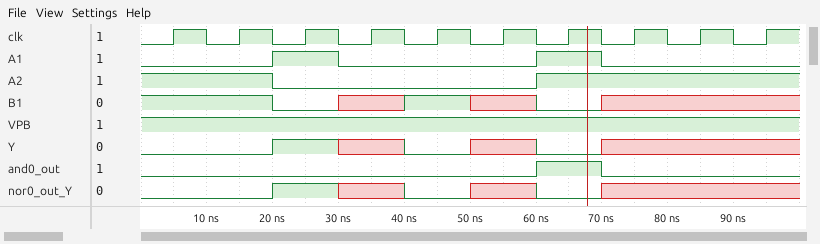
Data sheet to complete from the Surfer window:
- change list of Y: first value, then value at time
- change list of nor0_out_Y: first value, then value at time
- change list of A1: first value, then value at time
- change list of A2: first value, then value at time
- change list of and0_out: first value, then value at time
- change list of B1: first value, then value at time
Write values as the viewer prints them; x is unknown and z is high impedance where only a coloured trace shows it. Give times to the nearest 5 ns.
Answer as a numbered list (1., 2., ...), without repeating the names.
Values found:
1. 0, 1 at 20 ns, x at 30 ns, 0 at 40 ns, x at 50 ns, 0 at 60 ns, x at 70 ns
2. 0, 1 at 20 ns, x at 30 ns, 0 at 40 ns, x at 50 ns, 0 at 60 ns, x at 70 ns
3. 0, 1 at 20 ns, 0 at 30 ns, 1 at 60 ns, 0 at 70 ns
4. 1, 0 at 20 ns, 1 at 60 ns
5. 0, 1 at 60 ns, 0 at 70 ns
6. 1, 0 at 20 ns, x at 30 ns, 1 at 40 ns, x at 50 ns, 0 at 60 ns, x at 70 ns
